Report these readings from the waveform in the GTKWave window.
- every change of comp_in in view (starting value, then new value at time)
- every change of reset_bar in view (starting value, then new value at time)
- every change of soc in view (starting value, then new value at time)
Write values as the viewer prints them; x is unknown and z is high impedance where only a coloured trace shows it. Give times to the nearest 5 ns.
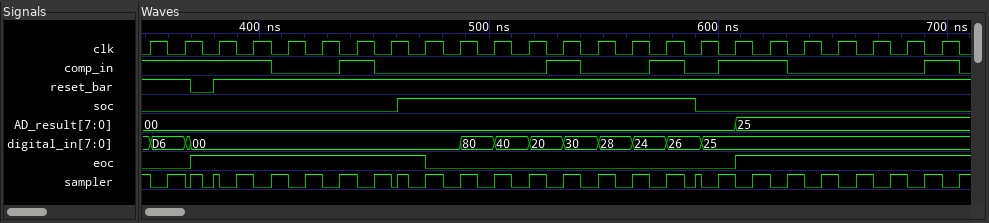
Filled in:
1, 0 at 405 ns, 1 at 435 ns, 0 at 450 ns, 1 at 525 ns, 0 at 540 ns, 1 at 570 ns, 0 at 585 ns, 1 at 600 ns, 0 at 630 ns, 1 at 690 ns, 0 at 705 ns
1, 0 at 370 ns, 1 at 380 ns
0, 1 at 460 ns, 0 at 590 ns
